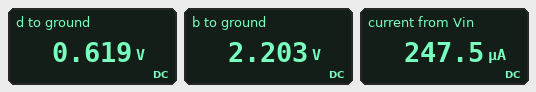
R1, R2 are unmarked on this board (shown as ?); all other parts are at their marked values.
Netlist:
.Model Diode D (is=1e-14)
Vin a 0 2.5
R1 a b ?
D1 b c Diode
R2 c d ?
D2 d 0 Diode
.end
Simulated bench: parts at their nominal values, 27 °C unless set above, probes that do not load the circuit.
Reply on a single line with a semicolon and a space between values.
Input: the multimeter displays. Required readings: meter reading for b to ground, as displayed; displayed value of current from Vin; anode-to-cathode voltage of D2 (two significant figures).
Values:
2.203 V; 247.5 µA; 620 mV
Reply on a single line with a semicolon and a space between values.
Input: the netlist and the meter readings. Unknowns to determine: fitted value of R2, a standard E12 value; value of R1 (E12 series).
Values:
3.9 kΩ; 1.2 kΩ
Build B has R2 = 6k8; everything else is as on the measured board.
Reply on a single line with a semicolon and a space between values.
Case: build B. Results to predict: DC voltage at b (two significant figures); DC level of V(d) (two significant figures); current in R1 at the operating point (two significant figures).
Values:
2.3 V; 610 mV; 160 µA
